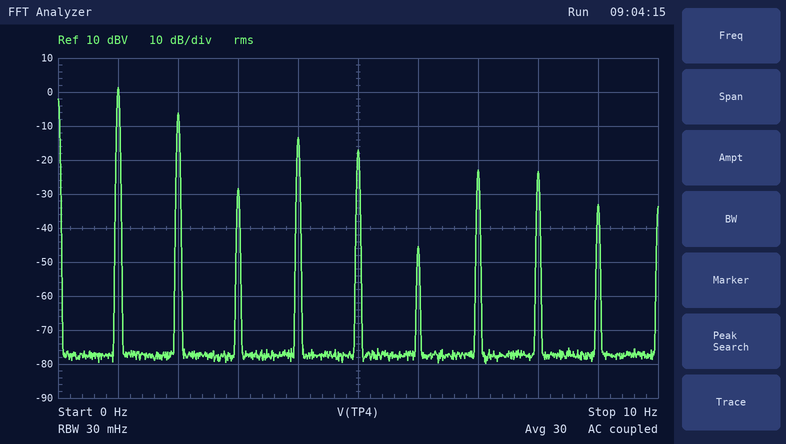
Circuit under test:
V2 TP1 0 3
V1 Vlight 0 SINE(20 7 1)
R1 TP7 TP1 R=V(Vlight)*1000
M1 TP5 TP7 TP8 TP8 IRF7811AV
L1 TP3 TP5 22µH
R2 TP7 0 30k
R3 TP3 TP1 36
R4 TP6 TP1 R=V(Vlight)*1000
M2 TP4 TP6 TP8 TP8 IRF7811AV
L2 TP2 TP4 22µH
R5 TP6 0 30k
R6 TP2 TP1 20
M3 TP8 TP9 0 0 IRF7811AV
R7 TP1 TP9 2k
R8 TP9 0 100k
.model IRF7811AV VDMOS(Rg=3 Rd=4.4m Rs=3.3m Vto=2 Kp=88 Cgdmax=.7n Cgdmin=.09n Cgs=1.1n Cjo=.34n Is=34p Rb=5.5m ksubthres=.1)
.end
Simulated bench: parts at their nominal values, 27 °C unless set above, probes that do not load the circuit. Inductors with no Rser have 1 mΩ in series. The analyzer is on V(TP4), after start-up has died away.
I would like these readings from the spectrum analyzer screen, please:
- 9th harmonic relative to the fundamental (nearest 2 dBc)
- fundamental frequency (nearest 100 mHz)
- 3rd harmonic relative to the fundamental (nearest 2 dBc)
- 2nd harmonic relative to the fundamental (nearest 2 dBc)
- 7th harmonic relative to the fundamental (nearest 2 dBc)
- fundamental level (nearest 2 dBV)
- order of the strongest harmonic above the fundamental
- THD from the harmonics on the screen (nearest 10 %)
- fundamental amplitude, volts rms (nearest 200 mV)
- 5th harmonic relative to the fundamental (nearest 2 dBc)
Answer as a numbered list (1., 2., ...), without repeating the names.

1. -34 dBc
2. 1.0 Hz
3. -30 dBc
4. -8 dBc
5. -24 dBc
6. 2 dBV
7. 2
8. 50 %
9. 1.2 V
10. -18 dBc
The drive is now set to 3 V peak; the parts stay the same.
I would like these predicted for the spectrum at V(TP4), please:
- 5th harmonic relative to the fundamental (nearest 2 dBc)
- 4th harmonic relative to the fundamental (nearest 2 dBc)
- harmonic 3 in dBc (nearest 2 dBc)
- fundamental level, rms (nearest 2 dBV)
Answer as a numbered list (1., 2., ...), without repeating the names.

1. -46 dBc
2. -30 dBc
3. -18 dBc
4. -10 dBV
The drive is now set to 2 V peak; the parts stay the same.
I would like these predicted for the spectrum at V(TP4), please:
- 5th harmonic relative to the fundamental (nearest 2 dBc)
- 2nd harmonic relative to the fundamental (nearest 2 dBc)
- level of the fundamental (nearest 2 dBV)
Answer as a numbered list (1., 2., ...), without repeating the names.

1. -58 dBc
2. -10 dBc
3. -16 dBV
